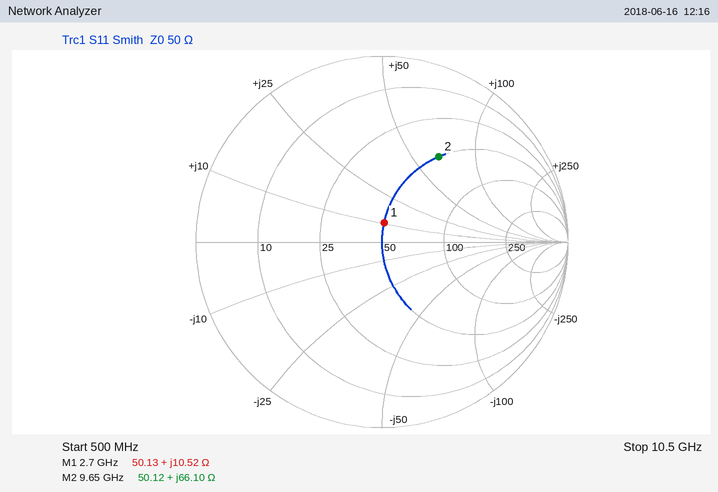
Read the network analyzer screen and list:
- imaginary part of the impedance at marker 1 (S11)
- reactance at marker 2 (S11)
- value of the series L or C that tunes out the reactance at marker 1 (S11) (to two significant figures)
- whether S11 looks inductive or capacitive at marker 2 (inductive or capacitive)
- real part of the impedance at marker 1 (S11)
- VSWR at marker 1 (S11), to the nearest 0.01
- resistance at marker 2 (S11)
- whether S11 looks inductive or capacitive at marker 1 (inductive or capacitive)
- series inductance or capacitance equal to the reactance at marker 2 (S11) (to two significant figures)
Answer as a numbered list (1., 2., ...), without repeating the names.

1. +10.52 Ω
2. +66.10 Ω
3. 5.6 pF
4. inductive
5. 50.13 Ω
6. 1.23
7. 50.12 Ω
8. inductive
9. 1.1 nH
